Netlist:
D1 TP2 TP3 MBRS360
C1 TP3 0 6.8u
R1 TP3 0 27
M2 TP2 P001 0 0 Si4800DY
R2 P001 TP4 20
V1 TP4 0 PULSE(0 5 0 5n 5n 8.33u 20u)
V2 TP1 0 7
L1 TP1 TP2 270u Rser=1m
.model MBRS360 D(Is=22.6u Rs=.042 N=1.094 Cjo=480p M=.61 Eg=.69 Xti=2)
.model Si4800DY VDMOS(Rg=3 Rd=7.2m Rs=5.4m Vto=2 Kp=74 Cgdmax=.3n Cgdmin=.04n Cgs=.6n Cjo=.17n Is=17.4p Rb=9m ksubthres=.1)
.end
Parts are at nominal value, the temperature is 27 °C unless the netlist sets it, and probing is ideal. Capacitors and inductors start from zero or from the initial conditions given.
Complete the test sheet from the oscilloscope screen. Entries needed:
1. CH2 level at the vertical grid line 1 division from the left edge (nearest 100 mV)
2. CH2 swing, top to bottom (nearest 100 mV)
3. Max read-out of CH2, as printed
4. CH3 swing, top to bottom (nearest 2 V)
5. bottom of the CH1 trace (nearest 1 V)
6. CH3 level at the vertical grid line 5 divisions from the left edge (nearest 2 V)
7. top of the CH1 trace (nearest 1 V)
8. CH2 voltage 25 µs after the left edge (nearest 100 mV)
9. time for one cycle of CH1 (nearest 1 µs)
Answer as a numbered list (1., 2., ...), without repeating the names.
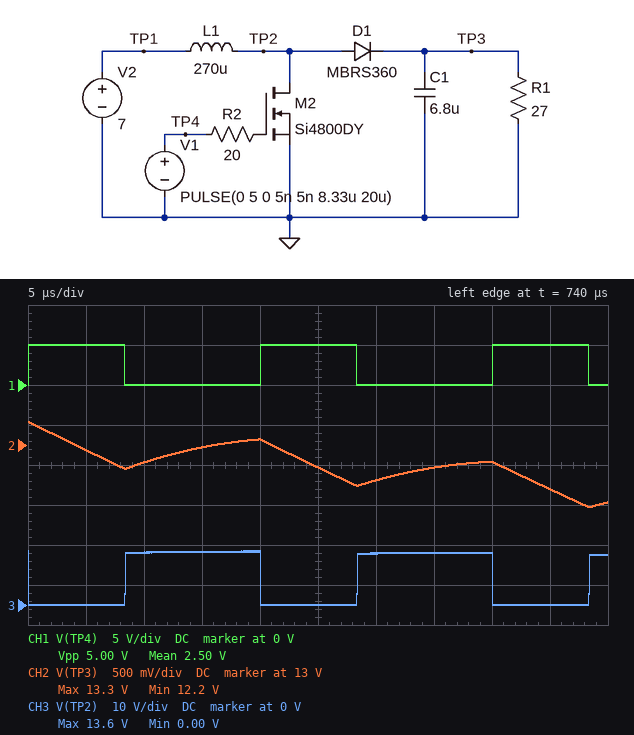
1. 12.9 V
2. 1.1 V
3. 13.3 V
4. 14 V
5. 0 V
6. 0 V
7. 5 V
8. 12.7 V
9. 20 µs
